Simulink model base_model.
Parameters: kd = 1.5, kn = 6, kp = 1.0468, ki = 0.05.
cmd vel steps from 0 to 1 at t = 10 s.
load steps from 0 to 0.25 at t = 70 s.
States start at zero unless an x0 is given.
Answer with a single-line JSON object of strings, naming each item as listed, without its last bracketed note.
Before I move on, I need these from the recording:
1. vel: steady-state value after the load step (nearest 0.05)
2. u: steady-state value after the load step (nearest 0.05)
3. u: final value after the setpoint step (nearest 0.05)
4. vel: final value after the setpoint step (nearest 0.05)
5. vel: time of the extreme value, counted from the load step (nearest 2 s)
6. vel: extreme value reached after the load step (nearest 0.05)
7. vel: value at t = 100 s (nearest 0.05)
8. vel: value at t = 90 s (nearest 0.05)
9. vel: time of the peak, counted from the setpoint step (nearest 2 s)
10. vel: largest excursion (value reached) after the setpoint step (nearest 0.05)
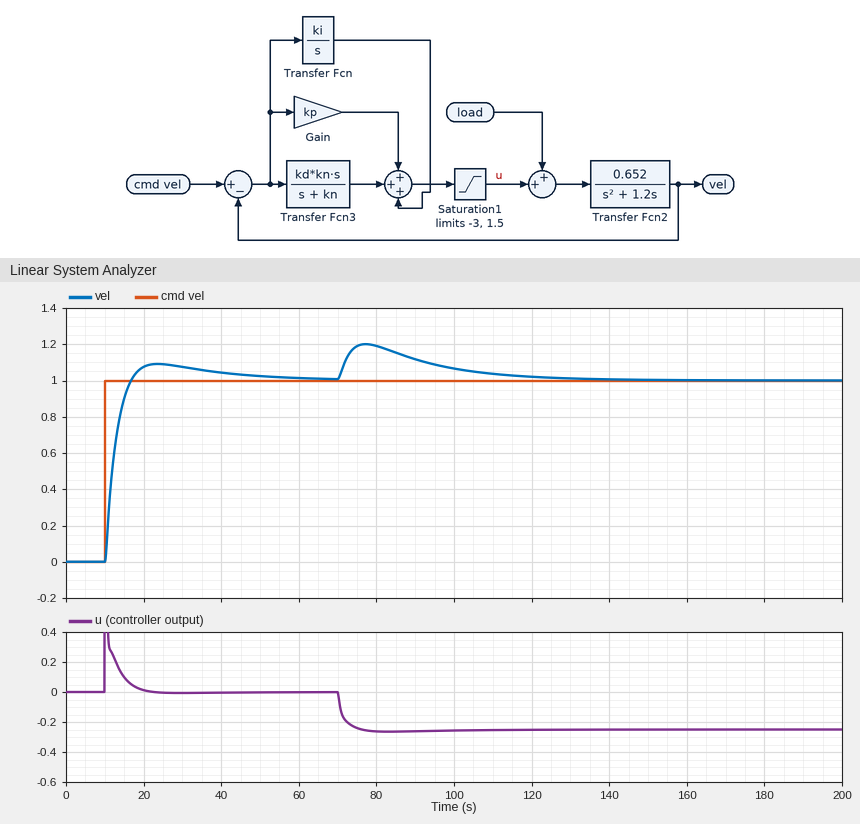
{"vel: steady-state value after the load step": "1.00", "u: steady-state value after the load step": "-0.25", "u: final value after the setpoint step": "0.00", "vel: final value after the setpoint step": "1.00", "vel: time of the extreme value, counted from the load step": "8 s", "vel: extreme value reached after the load step": "1.20", "vel: value at t = 100 s": "1.05", "vel: value at t = 90 s": "1.10", "vel: time of the peak, counted from the setpoint step": "14 s", "vel: largest excursion (value reached) after the setpoint step": "1.10"}
